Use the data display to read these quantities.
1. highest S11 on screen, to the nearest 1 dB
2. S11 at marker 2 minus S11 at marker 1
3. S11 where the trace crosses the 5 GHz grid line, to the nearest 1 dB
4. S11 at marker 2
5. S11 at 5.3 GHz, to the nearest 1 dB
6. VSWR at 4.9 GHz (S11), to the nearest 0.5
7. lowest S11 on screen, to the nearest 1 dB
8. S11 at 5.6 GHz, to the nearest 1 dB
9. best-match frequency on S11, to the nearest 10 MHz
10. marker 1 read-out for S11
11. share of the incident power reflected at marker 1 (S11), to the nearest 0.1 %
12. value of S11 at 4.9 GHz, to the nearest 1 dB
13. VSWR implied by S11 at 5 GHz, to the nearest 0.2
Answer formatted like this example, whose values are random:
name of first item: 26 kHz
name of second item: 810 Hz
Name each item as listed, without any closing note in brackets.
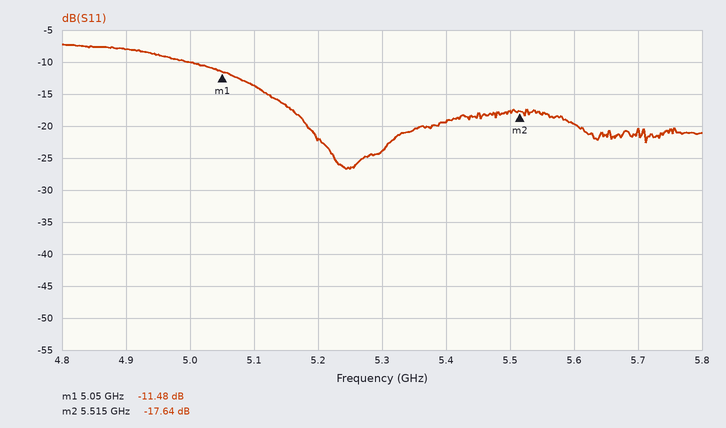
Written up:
highest S11 on screen, to the nearest 1 dB: -7 dB
S11 at marker 2 minus S11 at marker 1: -6.16 dB
S11 where the trace crosses the 5 GHz grid line, to the nearest 1 dB: -10 dB
S11 at marker 2: -17.64 dB
S11 at 5.3 GHz, to the nearest 1 dB: -24 dB
VSWR at 4.9 GHz (S11), to the nearest 0.5: 2.5
lowest S11 on screen, to the nearest 1 dB: -27 dB
S11 at 5.6 GHz, to the nearest 1 dB: -20 dB
best-match frequency on S11, to the nearest 10 MHz: 5.24 GHz
marker 1 read-out for S11: -11.48 dB
share of the incident power reflected at marker 1 (S11), to the nearest 0.1 %: 7.1 %
value of S11 at 4.9 GHz, to the nearest 1 dB: -8 dB
VSWR implied by S11 at 5 GHz, to the nearest 0.2: 2.0
